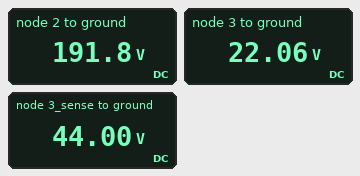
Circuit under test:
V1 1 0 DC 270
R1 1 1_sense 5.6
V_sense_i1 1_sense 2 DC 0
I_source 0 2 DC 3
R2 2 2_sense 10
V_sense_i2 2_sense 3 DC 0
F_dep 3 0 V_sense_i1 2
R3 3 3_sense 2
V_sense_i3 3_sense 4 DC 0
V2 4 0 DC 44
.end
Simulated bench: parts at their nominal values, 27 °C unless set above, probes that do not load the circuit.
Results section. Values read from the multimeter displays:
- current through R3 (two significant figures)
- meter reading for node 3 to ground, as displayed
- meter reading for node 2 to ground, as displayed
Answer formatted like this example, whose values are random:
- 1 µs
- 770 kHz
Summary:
- 11 A
- 22.06 V
- 191.8 V
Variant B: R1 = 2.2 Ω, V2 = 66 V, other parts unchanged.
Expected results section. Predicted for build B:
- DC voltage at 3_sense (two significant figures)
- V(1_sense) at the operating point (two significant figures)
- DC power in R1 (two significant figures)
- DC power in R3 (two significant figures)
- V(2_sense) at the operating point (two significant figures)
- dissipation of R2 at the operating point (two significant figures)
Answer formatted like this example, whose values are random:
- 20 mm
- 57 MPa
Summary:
- 66 V
- 230 V
- 600 W
- 360 W
- 39 V
- 3.8 kW
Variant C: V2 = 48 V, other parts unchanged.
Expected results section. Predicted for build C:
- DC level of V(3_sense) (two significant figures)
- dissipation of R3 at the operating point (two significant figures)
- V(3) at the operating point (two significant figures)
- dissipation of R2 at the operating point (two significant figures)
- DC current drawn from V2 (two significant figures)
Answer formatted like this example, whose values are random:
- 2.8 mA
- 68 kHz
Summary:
- 48 V
- 230 W
- 27 V
- 2.8 kW
- 11 A
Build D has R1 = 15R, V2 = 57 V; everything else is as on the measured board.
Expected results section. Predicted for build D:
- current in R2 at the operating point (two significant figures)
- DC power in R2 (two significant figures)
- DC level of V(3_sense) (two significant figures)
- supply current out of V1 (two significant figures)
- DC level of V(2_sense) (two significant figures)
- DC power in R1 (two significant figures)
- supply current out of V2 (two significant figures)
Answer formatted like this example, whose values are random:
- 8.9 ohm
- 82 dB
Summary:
- 11 A
- 1.1 kW
- 57 V
- 7.7 A
- 48 V
- 890 W
- 4.7 A
